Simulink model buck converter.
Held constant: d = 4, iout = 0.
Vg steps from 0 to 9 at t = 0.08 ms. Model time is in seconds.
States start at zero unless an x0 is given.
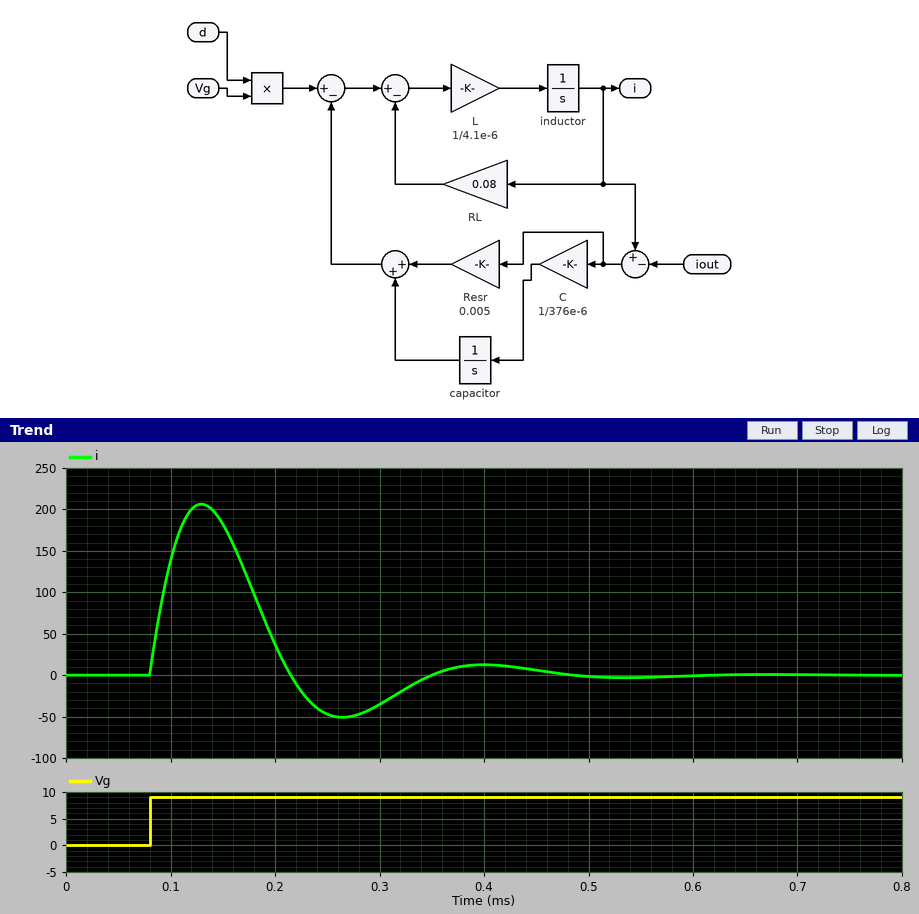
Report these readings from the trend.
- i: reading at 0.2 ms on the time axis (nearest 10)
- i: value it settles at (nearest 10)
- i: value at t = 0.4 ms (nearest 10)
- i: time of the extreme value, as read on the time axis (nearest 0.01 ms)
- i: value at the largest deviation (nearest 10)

40
0
10
0.13 ms
210
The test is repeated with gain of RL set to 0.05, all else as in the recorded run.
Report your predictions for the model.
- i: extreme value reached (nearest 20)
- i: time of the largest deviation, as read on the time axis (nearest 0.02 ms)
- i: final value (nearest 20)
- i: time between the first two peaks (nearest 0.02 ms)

240
0.14 ms
0
0.26 ms
